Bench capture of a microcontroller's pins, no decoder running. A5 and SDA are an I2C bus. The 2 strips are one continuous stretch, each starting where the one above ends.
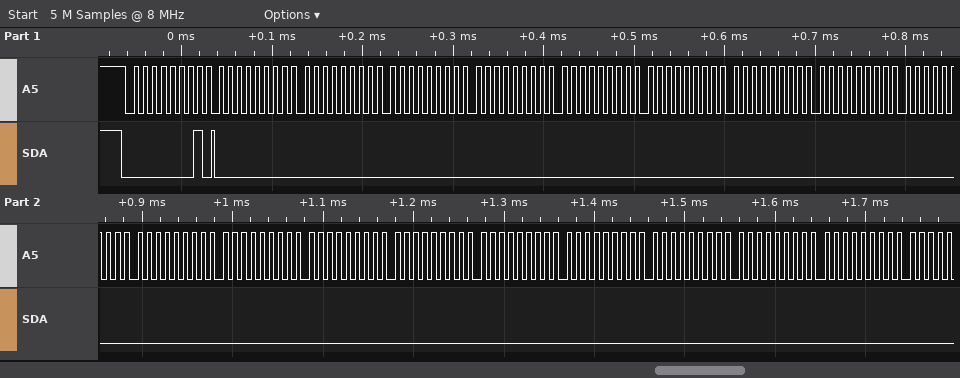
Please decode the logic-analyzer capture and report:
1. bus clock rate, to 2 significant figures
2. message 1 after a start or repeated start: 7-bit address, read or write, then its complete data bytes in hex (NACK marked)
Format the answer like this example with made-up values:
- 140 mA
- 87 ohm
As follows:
- 100 kHz
- 0x00 read: 00 00 00 00 00 00 00 00 00 00 00 00 00 00 00 00 00 00
